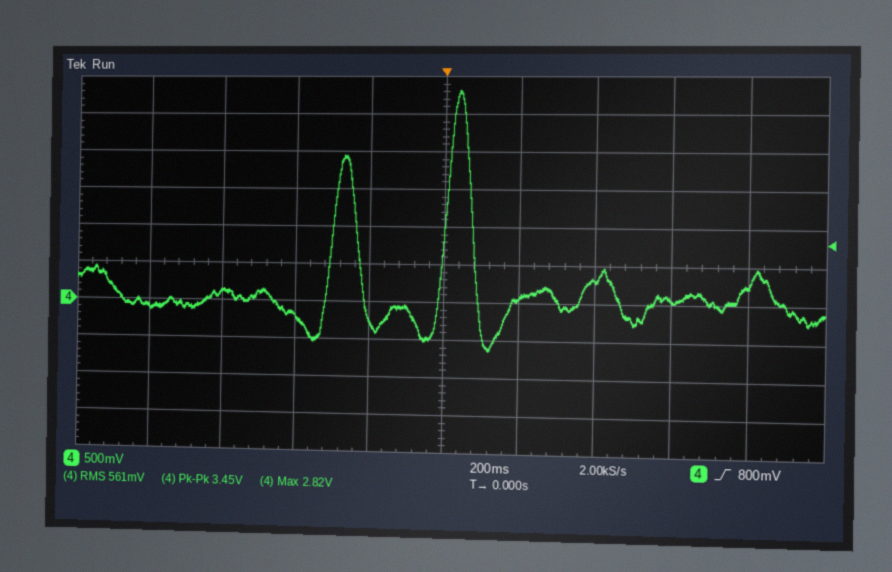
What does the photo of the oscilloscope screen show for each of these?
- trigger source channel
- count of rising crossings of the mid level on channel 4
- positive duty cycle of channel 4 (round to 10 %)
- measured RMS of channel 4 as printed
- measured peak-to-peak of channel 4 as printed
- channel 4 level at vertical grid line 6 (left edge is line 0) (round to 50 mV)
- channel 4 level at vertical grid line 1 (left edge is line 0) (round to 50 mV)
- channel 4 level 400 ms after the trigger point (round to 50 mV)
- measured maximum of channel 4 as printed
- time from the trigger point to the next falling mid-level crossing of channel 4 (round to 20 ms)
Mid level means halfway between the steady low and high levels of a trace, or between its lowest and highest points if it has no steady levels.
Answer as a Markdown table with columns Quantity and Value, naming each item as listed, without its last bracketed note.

| Quantity | Value |
|---|---|
| trigger source channel | channel 4 |
| count of rising crossings of the mid level on channel 4 | 2 |
| positive duty cycle of channel 4 | 20 % |
| measured RMS of channel 4 as printed | 561 mV |
| measured peak-to-peak of channel 4 as printed | 3.45 V |
| channel 4 level at vertical grid line 6 (left edge is line 0) | 50 mV |
| channel 4 level at vertical grid line 1 (left edge is line 0) | -100 mV |
| channel 4 level 400 ms after the trigger point | 300 mV |
| measured maximum of channel 4 as printed | 2.82 V |
| time from the trigger point to the next falling mid-level crossing of channel 4 | 80 ms |
